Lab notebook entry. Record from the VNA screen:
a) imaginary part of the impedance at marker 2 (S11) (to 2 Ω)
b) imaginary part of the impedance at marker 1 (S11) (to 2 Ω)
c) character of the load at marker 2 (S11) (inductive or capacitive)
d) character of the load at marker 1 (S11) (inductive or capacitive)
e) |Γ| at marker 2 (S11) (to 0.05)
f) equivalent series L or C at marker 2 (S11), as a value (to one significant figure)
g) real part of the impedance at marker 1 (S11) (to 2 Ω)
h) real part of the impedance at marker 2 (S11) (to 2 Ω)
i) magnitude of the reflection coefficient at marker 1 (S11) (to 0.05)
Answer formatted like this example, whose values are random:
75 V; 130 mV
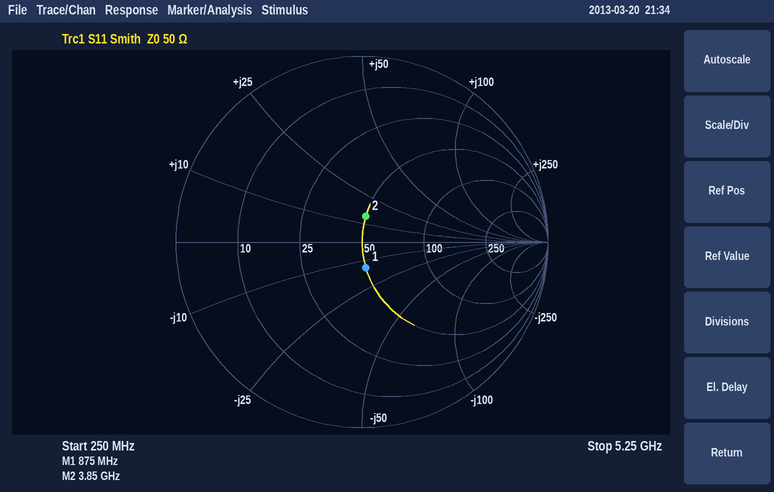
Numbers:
+14 Ω; -14 Ω; inductive; capacitive; 0.15; 600 pH; 50 Ω; 50 Ω; 0.15
